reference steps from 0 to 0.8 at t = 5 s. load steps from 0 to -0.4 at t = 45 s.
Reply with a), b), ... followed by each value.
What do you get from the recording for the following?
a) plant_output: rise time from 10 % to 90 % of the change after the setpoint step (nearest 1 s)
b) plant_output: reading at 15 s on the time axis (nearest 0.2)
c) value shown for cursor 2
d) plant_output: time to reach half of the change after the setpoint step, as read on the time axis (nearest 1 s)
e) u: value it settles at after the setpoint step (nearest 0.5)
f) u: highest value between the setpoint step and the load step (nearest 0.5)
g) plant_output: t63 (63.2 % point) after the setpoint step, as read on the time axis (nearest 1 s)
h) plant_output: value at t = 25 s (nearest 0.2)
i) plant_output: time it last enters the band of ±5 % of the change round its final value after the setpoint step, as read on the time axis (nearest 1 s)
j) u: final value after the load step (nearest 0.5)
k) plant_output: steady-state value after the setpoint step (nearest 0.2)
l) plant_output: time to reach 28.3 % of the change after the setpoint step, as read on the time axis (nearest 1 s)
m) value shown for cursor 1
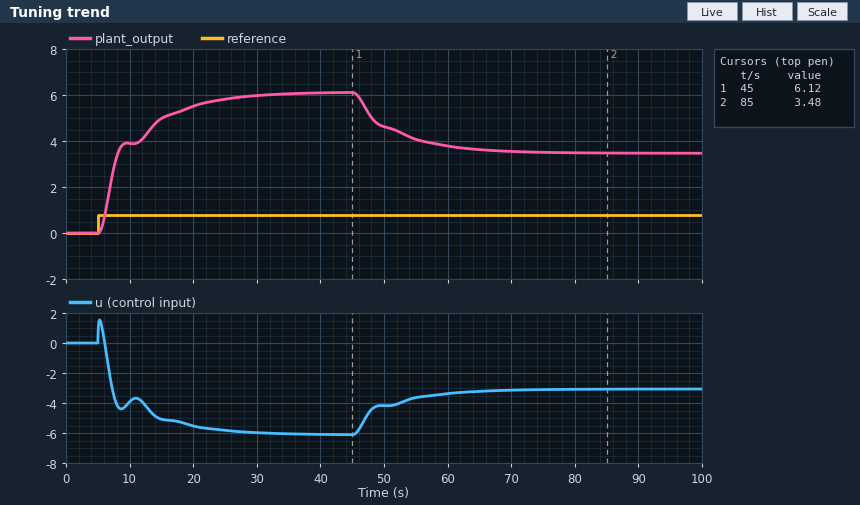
a) 14 s
b) 5.0
c) 3.48
d) 8 s
e) -6.0
f) 1.5
g) 9 s
h) 5.8
i) 25 s
j) -3.0
k) 6.2
l) 7 s
m) 6.12
